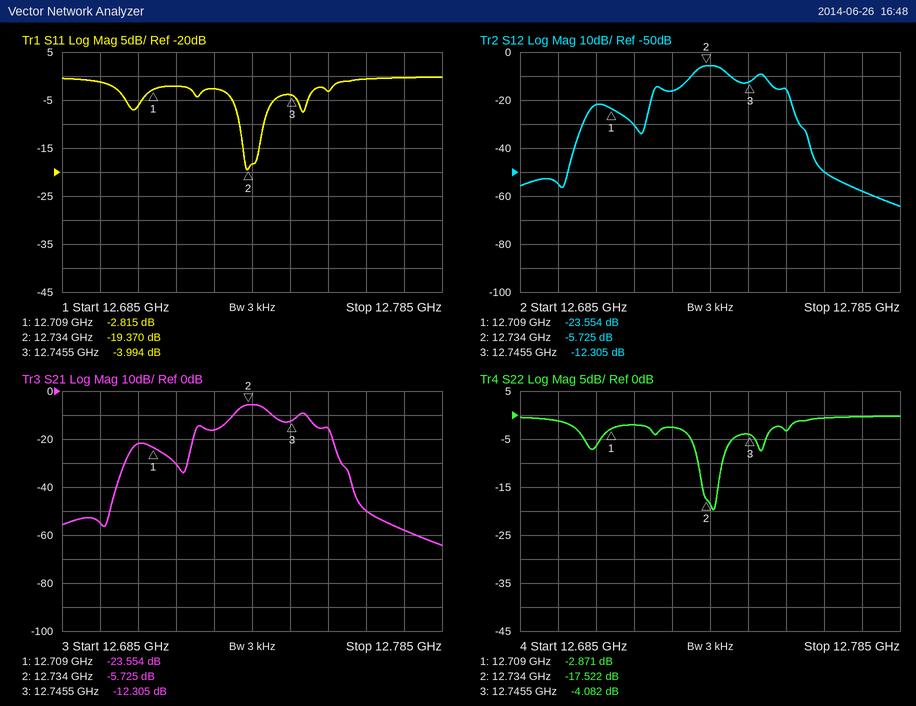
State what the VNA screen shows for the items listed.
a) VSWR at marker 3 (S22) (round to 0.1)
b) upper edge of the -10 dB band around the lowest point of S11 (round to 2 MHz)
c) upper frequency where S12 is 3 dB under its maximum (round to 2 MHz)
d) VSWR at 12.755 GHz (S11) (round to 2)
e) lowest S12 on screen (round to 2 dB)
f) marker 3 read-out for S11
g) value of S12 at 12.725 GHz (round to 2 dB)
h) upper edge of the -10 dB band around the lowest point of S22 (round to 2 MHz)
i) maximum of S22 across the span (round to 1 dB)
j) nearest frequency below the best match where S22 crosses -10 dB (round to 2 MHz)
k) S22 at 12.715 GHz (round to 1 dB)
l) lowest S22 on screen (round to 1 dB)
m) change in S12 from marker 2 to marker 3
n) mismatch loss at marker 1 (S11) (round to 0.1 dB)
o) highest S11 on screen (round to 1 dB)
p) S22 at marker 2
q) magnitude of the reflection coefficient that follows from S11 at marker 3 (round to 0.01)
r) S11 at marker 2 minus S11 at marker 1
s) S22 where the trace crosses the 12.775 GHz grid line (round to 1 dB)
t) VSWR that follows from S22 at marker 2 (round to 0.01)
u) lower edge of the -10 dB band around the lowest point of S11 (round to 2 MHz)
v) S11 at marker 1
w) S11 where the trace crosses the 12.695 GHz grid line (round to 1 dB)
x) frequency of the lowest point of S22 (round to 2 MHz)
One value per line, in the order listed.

4.3
12.738 GHz
12.740 GHz
6
-64 dB
-3.994 dB
-16 dB
12.738 GHz
0 dB
12.732 GHz
-2 dB
-20 dB
-6.580 dB
3.2 dB
0 dB
-17.522 dB
0.63
-16.555 dB
0 dB
1.31
12.732 GHz
-2.815 dB
-1 dB
12.736 GHz
